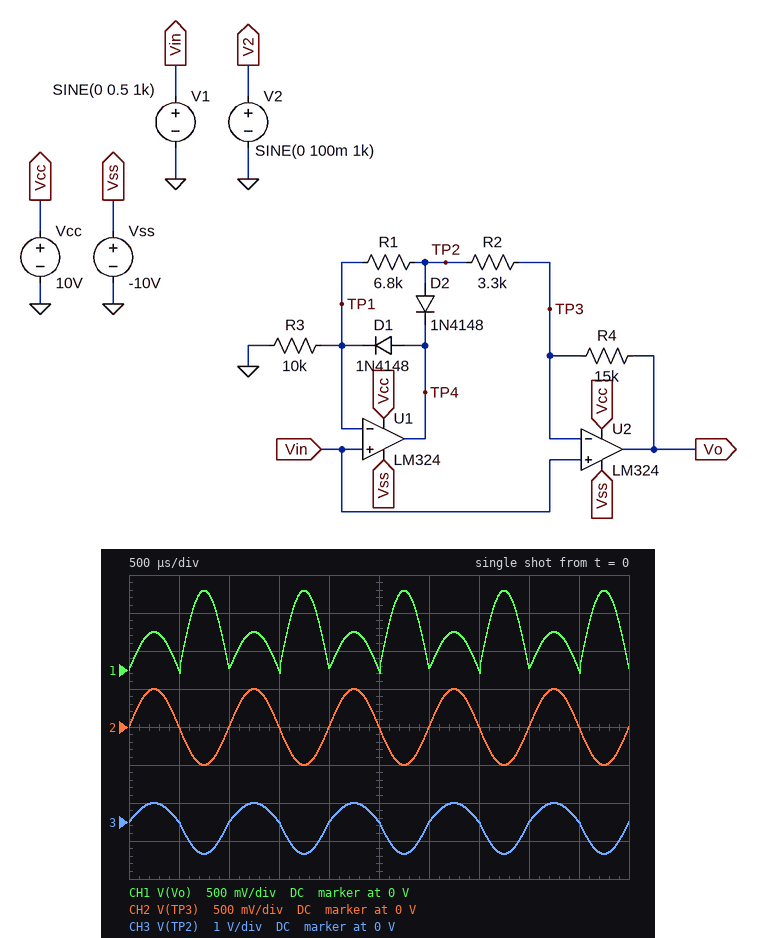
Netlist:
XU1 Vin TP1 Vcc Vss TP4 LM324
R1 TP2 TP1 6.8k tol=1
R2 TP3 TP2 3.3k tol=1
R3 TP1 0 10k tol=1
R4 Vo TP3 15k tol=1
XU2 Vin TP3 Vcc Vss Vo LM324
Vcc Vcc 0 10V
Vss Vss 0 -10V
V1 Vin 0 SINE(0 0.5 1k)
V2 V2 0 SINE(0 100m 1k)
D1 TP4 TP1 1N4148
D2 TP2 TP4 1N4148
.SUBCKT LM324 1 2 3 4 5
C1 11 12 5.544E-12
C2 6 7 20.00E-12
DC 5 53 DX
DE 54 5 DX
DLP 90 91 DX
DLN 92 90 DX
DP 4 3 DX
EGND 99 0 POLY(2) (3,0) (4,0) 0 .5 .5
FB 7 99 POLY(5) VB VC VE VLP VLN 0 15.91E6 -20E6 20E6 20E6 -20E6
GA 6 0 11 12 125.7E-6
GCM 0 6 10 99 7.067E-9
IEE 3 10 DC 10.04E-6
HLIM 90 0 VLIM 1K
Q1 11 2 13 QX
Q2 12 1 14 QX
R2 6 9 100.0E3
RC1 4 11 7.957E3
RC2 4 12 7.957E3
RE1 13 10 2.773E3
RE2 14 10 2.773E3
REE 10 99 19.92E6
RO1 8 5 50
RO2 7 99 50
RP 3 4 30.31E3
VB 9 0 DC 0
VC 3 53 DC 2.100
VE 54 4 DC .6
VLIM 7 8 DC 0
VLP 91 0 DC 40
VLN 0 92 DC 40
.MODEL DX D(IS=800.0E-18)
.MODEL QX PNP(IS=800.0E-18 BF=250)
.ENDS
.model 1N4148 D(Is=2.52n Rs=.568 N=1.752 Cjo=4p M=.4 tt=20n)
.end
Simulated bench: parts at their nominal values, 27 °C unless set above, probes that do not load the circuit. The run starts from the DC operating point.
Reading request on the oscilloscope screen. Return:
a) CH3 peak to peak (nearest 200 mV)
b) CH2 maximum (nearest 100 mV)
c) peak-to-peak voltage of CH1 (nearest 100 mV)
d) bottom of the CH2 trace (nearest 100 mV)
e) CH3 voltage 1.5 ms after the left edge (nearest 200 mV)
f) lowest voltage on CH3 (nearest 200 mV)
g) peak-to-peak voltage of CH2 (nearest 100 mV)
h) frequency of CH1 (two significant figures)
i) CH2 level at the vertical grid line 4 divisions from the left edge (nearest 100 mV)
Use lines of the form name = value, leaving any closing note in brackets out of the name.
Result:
CH3 peak to peak = 1.4 V
CH2 maximum = 500 mV
peak-to-peak voltage of CH1 = 1.1 V
bottom of the CH2 trace = -500 mV
CH3 voltage 1.5 ms after the left edge = 0 V
lowest voltage on CH3 = -800 mV
peak-to-peak voltage of CH2 = 1.0 V
frequency of CH1 = 1.0 kHz
CH2 level at the vertical grid line 4 divisions from the left edge = 0 V
